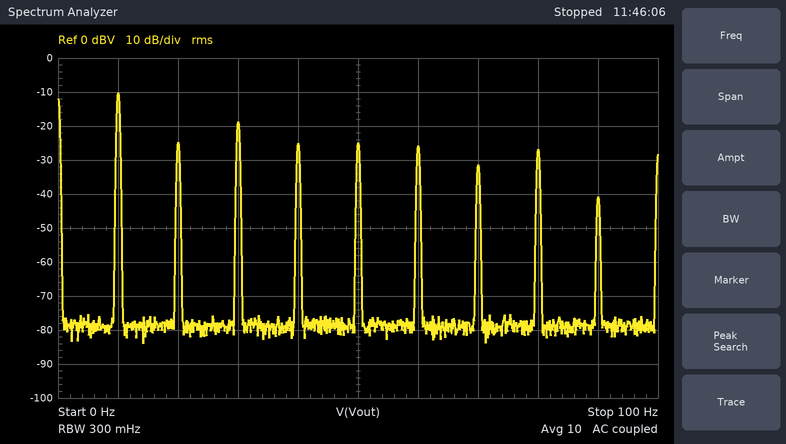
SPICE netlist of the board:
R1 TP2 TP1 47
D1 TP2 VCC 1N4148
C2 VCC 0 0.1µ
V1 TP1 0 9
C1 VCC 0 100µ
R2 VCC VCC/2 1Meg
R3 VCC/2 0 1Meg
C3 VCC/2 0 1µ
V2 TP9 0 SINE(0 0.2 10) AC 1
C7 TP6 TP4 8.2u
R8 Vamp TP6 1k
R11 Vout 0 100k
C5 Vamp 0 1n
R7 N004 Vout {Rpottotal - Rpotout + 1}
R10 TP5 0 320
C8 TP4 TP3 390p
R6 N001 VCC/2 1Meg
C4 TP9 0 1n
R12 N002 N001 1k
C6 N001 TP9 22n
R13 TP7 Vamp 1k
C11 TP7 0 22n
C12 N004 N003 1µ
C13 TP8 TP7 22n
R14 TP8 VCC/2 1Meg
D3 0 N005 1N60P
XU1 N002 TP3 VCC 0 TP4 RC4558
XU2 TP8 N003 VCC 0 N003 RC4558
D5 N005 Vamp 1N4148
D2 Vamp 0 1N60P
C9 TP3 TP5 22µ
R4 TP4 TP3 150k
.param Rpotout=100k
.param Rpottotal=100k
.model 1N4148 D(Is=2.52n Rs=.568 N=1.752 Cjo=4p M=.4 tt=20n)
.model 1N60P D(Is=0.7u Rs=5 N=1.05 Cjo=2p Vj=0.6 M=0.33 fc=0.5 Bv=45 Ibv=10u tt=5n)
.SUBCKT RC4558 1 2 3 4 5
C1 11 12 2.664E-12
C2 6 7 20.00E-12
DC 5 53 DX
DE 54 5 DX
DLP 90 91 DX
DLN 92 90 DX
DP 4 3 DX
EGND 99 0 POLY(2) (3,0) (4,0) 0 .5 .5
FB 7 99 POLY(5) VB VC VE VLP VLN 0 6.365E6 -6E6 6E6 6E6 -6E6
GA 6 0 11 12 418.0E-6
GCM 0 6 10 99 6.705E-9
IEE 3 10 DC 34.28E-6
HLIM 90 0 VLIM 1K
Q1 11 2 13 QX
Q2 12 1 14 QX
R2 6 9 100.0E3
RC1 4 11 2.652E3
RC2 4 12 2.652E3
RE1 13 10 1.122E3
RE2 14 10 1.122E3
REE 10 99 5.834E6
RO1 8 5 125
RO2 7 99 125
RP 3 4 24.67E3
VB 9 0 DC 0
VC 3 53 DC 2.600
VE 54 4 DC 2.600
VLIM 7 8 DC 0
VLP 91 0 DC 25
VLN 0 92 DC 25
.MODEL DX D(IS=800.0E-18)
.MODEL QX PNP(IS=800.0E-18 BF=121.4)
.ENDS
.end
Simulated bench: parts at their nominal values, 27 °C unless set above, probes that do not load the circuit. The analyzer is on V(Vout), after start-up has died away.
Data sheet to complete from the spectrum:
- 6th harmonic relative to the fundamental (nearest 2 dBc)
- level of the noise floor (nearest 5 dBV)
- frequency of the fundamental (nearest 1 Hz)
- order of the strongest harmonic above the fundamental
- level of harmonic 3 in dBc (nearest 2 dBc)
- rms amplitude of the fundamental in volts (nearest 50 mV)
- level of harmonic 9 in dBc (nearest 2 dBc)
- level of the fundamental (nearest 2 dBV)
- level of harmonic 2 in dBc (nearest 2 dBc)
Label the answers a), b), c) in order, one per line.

a) -16 dBc
b) -80 dBV
c) 10 Hz
d) 3
e) -8 dBc
f) 300 mV
g) -30 dBc
h) -10 dBV
i) -14 dBc
